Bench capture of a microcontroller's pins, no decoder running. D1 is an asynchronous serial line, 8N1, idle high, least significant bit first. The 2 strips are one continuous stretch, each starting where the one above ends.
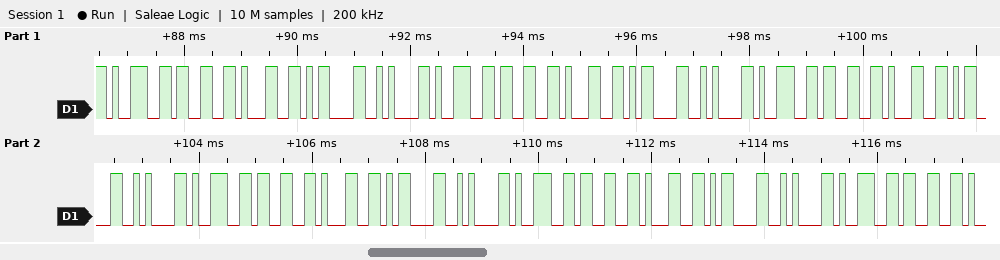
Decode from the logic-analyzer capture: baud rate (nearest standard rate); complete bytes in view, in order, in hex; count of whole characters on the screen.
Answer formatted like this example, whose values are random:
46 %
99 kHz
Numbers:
9600 baud
39 33 31 0D 0A 39 33 31 0D 0A 39 33 31 0D 0A 39 33 31 0D 0A 39 33 31 0D 0A 39 33
27
